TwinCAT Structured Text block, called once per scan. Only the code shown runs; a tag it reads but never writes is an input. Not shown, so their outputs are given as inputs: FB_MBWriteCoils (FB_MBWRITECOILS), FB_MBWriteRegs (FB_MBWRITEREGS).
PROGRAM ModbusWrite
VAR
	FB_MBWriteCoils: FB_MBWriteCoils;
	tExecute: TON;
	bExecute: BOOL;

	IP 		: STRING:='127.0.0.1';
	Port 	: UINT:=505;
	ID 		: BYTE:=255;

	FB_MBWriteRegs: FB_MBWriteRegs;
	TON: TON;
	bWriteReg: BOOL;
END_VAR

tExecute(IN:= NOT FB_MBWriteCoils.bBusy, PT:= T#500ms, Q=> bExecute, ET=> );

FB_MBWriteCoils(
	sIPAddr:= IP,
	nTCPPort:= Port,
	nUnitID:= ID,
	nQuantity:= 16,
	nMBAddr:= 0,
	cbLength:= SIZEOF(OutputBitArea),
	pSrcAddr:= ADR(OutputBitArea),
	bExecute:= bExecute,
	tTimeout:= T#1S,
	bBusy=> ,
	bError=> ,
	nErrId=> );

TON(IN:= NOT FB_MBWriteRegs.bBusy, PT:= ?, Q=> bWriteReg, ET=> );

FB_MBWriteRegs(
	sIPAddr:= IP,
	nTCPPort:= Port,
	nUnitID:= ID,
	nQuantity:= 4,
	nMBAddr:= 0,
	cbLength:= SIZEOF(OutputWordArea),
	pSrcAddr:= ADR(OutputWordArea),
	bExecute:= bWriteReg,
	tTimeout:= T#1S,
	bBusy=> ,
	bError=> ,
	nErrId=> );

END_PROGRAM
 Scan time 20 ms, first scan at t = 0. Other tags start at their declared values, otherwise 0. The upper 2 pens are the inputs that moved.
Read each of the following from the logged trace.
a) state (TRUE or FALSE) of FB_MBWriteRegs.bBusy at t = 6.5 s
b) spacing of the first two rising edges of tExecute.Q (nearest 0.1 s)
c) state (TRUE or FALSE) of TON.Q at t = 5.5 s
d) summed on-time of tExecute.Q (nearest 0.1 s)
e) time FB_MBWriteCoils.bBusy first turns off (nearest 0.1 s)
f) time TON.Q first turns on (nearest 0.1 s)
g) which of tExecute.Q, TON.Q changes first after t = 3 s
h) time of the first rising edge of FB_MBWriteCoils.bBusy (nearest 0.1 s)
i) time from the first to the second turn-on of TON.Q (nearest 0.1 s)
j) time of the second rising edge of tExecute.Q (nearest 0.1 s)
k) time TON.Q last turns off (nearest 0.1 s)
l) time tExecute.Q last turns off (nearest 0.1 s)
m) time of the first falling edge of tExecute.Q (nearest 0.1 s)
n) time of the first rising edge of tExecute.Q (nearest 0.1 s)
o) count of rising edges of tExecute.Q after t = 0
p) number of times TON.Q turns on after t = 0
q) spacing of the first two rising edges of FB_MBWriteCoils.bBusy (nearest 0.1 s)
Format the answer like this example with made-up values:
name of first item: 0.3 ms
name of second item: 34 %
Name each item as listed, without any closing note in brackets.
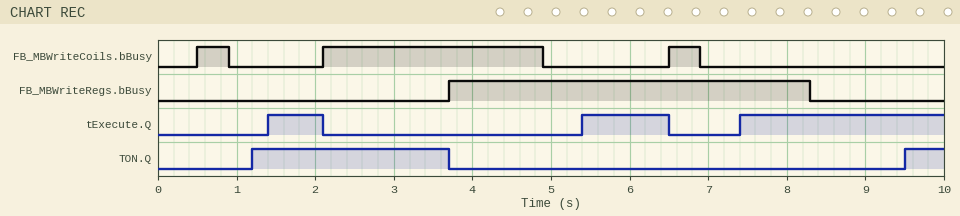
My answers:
state (TRUE or FALSE) of FB_MBWriteRegs.bBusy at t = 6.5 s: TRUE
spacing of the first two rising edges of tExecute.Q: 4.0 s
state (TRUE or FALSE) of TON.Q at t = 5.5 s: FALSE
summed on-time of tExecute.Q: 4.4 s
time FB_MBWriteCoils.bBusy first turns off: 0.9 s
time TON.Q first turns on: 1.2 s
which of tExecute.Q, TON.Q changes first after t = 3 s: TON.Q
time of the first rising edge of FB_MBWriteCoils.bBusy: 0.5 s
time from the first to the second turn-on of TON.Q: 8.3 s
time of the second rising edge of tExecute.Q: 5.4 s
time TON.Q last turns off: 3.7 s
time tExecute.Q last turns off: 6.5 s
time of the first falling edge of tExecute.Q: 2.1 s
time of the first rising edge of tExecute.Q: 1.4 s
count of rising edges of tExecute.Q after t = 0: 3
number of times TON.Q turns on after t = 0: 2
spacing of the first two rising edges of FB_MBWriteCoils.bBusy: 1.6 s
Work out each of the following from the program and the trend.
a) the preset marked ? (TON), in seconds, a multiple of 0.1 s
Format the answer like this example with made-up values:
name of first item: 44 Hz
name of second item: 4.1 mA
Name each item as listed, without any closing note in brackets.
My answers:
the preset marked ? (TON), in seconds, a multiple of 0.1 s: 1.2 s
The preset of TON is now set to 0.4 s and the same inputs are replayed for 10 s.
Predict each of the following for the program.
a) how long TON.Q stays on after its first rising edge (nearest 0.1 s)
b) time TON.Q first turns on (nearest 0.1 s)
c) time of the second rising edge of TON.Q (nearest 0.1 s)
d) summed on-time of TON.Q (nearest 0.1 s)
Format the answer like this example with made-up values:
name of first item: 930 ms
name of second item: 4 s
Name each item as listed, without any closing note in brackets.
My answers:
how long TON.Q stays on after its first rising edge: 3.3 s
time TON.Q first turns on: 0.4 s
time of the second rising edge of TON.Q: 8.7 s
summed on-time of TON.Q: 4.6 s
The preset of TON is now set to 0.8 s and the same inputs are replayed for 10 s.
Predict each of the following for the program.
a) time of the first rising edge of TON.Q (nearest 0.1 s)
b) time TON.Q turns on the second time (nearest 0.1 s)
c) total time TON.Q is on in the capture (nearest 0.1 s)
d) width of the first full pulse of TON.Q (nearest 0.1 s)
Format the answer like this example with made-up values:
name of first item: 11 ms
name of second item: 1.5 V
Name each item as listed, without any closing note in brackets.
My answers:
time of the first rising edge of TON.Q: 0.8 s
time TON.Q turns on the second time: 9.1 s
total time TON.Q is on in the capture: 3.8 s
width of the first full pulse of TON.Q: 2.9 s
